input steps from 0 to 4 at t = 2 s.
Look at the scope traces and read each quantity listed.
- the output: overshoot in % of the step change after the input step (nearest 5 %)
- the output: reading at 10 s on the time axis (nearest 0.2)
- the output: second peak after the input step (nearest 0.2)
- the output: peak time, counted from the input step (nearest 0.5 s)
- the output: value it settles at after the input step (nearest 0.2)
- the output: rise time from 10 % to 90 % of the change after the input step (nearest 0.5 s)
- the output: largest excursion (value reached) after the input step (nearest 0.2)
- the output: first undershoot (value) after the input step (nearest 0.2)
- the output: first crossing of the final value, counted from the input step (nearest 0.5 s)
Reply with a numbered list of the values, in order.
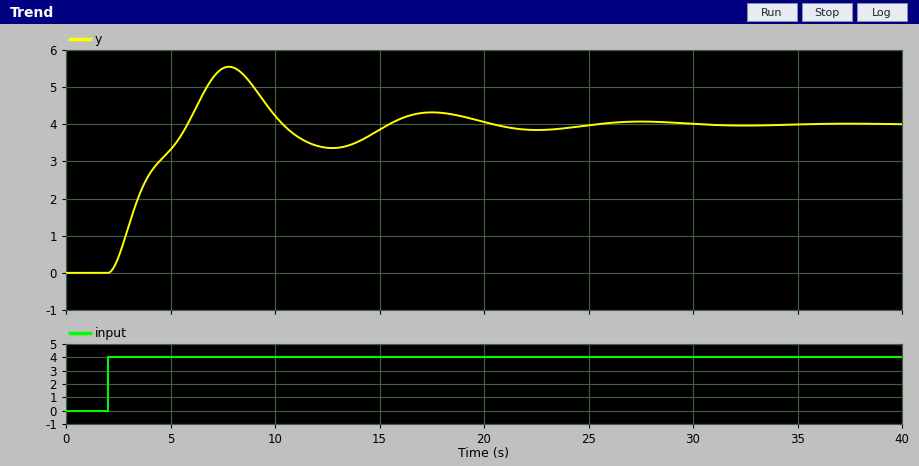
1. 40 %
2. 4.2
3. 4.4
4. 6.0 s
5. 4.0
6. 3.0 s
7. 5.6
8. 3.4
9. 4.0 s
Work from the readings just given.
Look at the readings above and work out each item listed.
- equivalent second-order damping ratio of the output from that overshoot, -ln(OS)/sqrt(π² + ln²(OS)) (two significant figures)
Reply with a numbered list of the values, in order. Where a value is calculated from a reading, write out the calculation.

1. ln(0.4) = -0.916; 0.916 / sqrt(9.870 + 0.840) = 0.28
